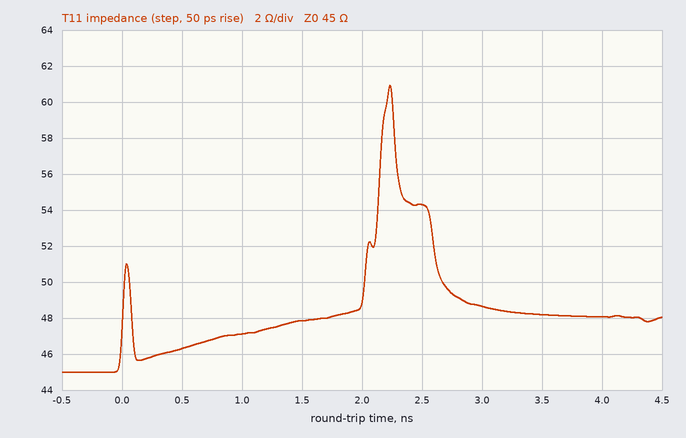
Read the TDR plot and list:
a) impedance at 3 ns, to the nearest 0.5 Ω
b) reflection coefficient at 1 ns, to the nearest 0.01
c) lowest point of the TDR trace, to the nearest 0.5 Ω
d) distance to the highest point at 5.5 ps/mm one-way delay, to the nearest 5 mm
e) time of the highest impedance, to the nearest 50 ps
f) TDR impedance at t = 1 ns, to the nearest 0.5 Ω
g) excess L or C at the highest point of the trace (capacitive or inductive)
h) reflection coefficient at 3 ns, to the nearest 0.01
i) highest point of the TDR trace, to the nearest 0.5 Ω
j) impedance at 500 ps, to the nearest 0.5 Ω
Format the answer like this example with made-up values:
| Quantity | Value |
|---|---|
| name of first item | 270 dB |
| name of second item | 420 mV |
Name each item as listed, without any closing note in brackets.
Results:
| Quantity | Value |
|---|---|
| impedance at 3 ns, to the nearest 0.5 Ω | 48.5 Ω |
| reflection coefficient at 1 ns, to the nearest 0.01 | +0.02 |
| lowest point of the TDR trace, to the nearest 0.5 Ω | 45.0 Ω |
| distance to the highest point at 5.5 ps/mm one-way delay, to the nearest 5 mm | 205 mm |
| time of the highest impedance, to the nearest 50 ps | 2.25 ns |
| TDR impedance at t = 1 ns, to the nearest 0.5 Ω | 47.0 Ω |
| excess L or C at the highest point of the trace | inductive |
| reflection coefficient at 3 ns, to the nearest 0.01 | +0.04 |
| highest point of the TDR trace, to the nearest 0.5 Ω | 61.0 Ω |
| impedance at 500 ps, to the nearest 0.5 Ω | 46.5 Ω |
